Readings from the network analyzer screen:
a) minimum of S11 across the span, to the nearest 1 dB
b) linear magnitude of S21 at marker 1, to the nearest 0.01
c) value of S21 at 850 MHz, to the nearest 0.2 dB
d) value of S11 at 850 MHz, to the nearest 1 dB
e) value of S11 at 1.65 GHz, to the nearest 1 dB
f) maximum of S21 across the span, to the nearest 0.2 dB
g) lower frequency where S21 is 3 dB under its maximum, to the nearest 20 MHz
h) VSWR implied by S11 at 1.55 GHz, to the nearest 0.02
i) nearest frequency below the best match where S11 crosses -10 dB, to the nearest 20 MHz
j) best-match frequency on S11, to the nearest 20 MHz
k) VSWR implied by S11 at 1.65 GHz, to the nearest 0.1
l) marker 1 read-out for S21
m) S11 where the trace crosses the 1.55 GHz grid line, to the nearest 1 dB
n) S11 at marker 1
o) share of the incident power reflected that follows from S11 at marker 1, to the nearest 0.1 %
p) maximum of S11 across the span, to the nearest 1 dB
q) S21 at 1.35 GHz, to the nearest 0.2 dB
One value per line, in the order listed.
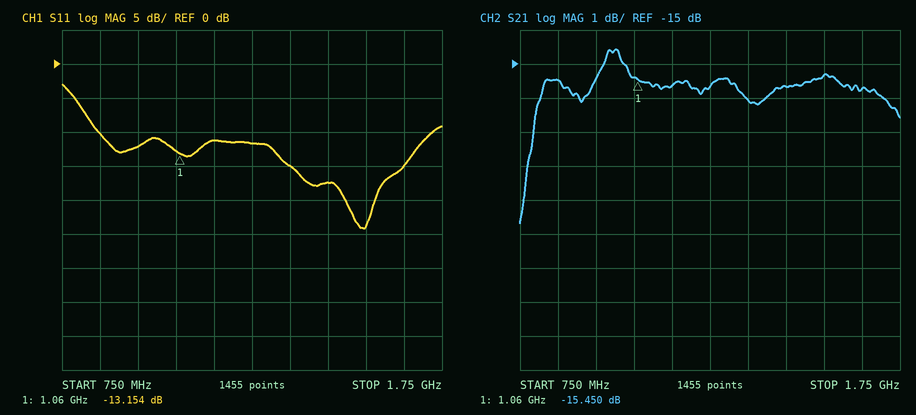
-24 dB
0.17
-15.4 dB
-10 dB
-15 dB
-14.6 dB
780 MHz
1.14
840 MHz
1.54 GHz
1.4
-15.450 dB
-24 dB
-13.154 dB
4.8 %
-3 dB
-16.0 dB
